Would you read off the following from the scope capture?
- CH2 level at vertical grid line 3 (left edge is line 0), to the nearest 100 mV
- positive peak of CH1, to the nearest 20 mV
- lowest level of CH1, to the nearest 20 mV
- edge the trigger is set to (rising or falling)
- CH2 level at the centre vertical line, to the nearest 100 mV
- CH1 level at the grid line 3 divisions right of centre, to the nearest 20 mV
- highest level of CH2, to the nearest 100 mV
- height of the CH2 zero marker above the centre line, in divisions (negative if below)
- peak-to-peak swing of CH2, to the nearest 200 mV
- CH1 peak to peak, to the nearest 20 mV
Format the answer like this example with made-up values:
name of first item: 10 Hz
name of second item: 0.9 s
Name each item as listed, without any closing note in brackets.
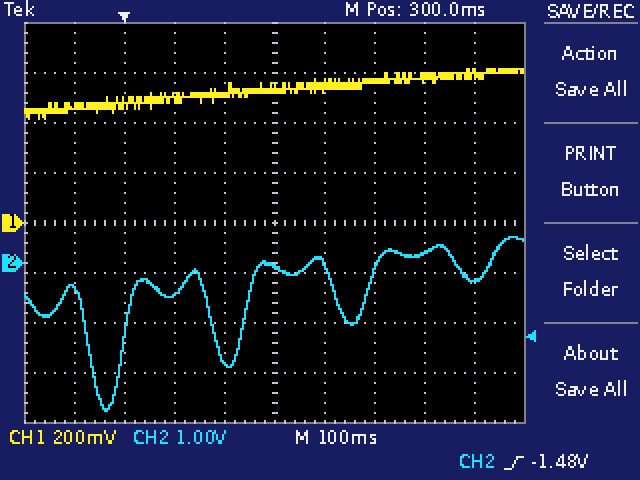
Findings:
CH2 level at vertical grid line 3 (left edge is line 0), to the nearest 100 mV: -600 mV
positive peak of CH1, to the nearest 20 mV: 620 mV
lowest level of CH1, to the nearest 20 mV: 420 mV
edge the trigger is set to: rising
CH2 level at the centre vertical line, to the nearest 100 mV: -100 mV
CH1 level at the grid line 3 divisions right of centre, to the nearest 20 mV: 580 mV
highest level of CH2, to the nearest 100 mV: 500 mV
height of the CH2 zero marker above the centre line, in divisions: -0.8 div
peak-to-peak swing of CH2, to the nearest 200 mV: 3.4 V
CH1 peak to peak, to the nearest 20 mV: 200 mV
